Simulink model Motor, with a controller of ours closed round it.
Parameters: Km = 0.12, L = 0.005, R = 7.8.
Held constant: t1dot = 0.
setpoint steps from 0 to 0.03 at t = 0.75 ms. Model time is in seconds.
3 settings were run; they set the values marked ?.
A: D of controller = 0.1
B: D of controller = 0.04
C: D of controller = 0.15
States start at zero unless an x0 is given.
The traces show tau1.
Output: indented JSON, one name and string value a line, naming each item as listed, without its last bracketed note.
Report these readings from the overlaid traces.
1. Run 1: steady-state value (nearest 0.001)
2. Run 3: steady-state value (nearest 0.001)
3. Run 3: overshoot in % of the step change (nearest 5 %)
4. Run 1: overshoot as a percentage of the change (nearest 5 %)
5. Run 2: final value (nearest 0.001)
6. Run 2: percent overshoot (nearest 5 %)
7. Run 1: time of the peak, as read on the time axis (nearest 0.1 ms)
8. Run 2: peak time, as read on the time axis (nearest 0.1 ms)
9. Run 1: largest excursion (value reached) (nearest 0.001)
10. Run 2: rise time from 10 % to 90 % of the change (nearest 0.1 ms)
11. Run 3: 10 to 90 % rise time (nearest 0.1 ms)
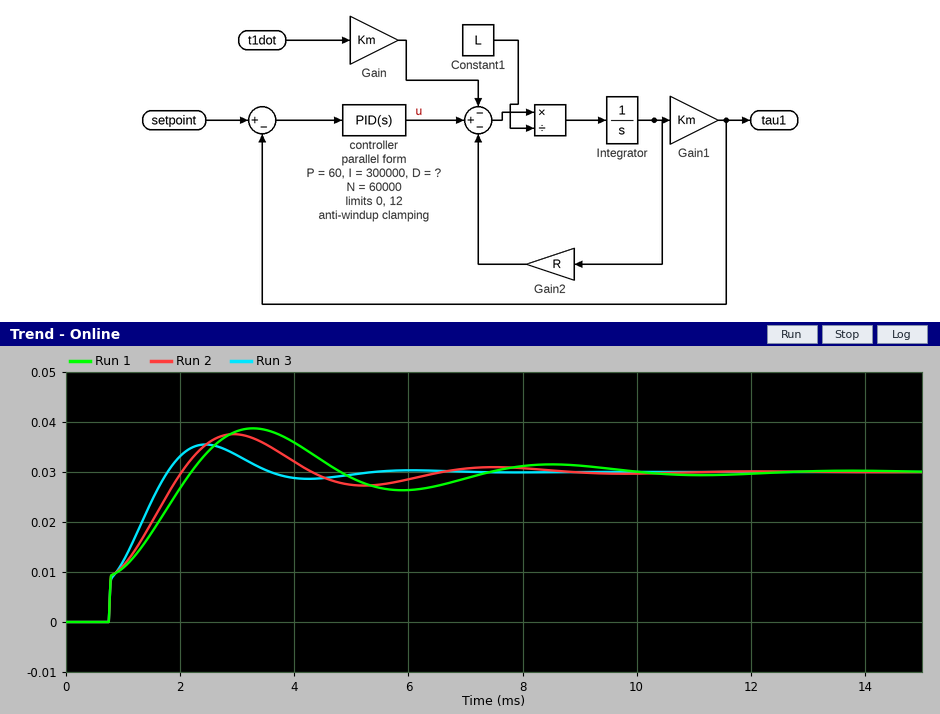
{
  "Run 1: steady-state value": "0.030",
  "Run 3: steady-state value": "0.030",
  "Run 3: overshoot in % of the step change": "20 %",
  "Run 1: overshoot as a percentage of the change": "30 %",
  "Run 2: final value": "0.030",
  "Run 2: percent overshoot": "25 %",
  "Run 1: time of the peak, as read on the time axis": "3.3 ms",
  "Run 2: peak time, as read on the time axis": "2.9 ms",
  "Run 1: largest excursion (value reached)": "0.039",
  "Run 2: rise time from 10 % to 90 % of the change": "1.1 ms",
  "Run 3: 10 to 90 % rise time": "0.9 ms"
}
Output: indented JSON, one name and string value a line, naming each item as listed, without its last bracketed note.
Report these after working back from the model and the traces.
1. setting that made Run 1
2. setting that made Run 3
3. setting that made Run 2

{
  "setting that made Run 1": "C",
  "setting that made Run 3": "B",
  "setting that made Run 2": "A"
}
